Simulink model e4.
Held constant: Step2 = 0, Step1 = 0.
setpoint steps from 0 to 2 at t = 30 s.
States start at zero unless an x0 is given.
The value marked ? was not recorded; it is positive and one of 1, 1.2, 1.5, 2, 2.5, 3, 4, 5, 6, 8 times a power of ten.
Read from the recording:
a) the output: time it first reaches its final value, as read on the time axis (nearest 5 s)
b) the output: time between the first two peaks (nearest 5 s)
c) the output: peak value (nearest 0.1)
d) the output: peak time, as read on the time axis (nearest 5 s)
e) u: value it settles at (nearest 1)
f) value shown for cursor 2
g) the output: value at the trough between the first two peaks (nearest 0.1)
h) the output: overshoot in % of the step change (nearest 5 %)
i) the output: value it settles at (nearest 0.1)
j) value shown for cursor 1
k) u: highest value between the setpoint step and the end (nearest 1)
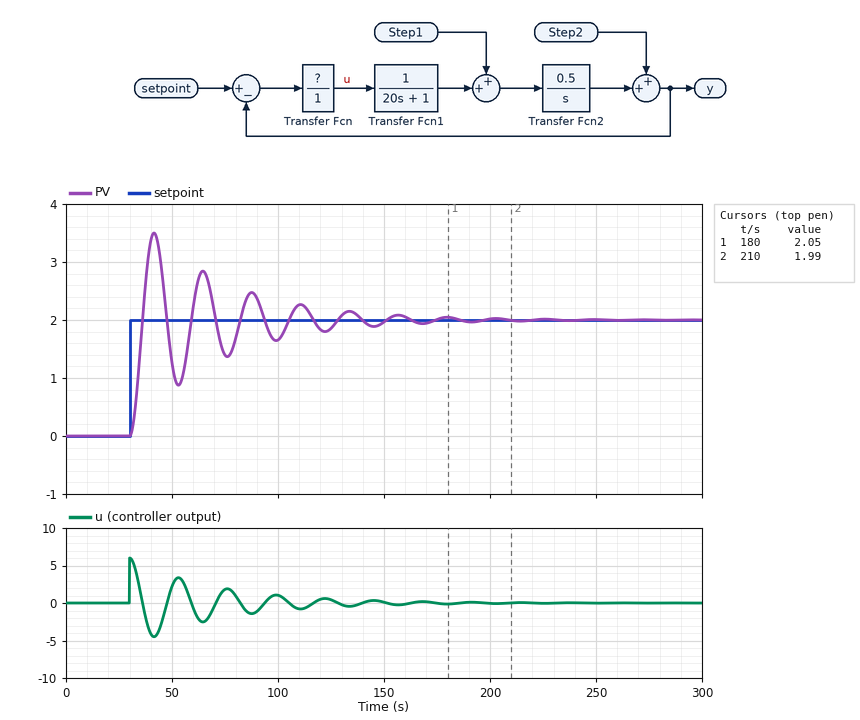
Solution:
35 s
25 s
3.5
40 s
0
1.99
0.9
75 %
2.0
2.05
6
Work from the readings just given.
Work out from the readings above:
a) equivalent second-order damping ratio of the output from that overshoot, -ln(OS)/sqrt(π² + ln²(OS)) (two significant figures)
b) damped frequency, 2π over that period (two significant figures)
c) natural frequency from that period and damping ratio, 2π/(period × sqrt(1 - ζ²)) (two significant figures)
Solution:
0.091
0.25 rad/s
0.25 rad/s
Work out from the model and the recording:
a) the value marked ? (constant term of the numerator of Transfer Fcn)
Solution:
3
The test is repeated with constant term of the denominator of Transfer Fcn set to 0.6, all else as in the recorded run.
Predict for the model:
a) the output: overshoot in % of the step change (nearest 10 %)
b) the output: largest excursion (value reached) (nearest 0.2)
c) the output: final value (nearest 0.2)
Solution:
80 %
3.6
2.0
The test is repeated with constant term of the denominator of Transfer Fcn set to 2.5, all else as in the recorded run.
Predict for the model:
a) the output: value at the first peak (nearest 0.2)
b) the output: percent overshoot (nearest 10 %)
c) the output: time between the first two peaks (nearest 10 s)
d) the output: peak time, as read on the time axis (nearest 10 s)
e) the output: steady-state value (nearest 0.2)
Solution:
3.2
60 %
40 s
50 s
2.0
